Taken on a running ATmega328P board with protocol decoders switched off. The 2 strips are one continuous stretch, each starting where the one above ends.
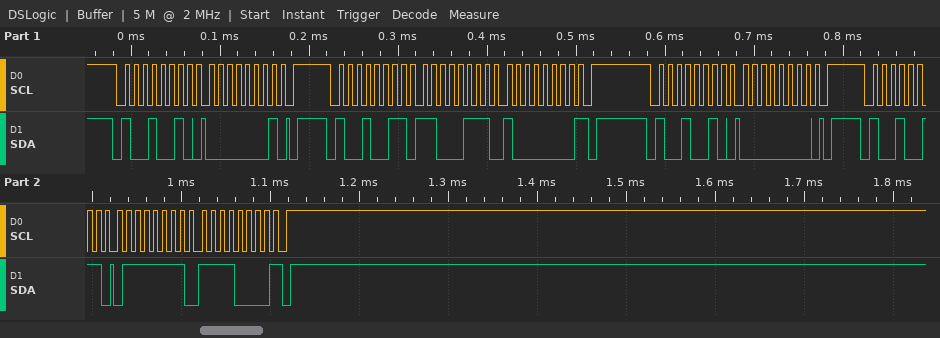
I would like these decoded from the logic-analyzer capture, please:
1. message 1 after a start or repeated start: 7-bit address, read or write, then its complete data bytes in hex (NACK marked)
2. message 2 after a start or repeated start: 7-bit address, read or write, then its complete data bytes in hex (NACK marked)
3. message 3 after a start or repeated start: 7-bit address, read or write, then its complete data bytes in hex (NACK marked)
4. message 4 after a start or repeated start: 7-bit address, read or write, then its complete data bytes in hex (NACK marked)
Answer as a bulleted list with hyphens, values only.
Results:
- 0x49 write: 01
- 0x49 read: C7 80 NACK
- 0x49 write: 00
- 0x49 read: 7F F0 NACK
